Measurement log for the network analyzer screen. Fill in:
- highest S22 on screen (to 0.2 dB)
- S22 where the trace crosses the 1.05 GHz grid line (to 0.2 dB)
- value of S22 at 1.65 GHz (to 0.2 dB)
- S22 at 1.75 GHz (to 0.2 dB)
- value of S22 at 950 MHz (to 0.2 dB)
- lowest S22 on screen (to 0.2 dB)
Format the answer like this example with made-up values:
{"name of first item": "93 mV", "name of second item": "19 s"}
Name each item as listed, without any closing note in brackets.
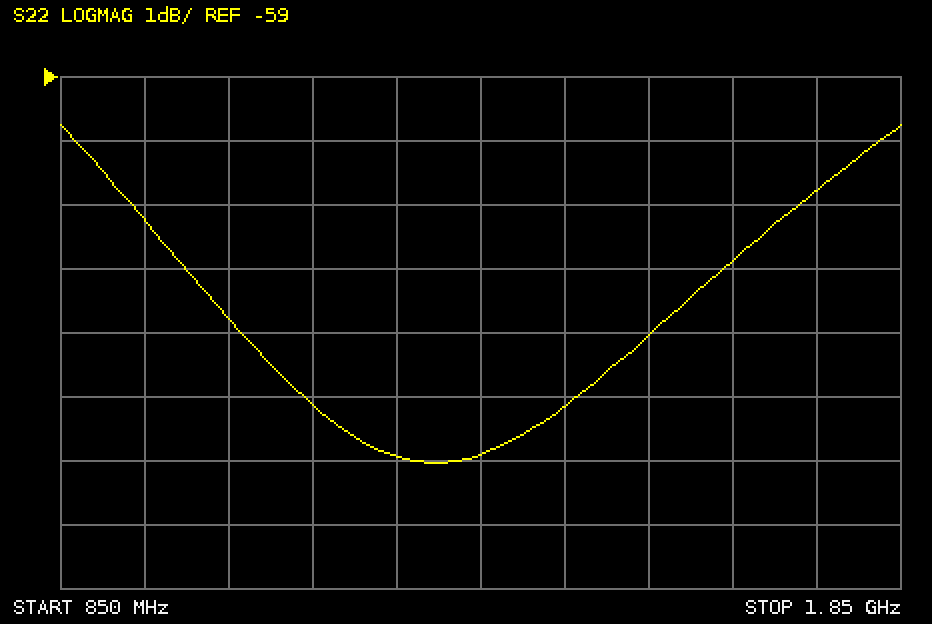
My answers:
{"highest S22 on screen": "-59.8 dB", "S22 where the trace crosses the 1.05 GHz grid line": "-62.8 dB", "value of S22 at 1.65 GHz": "-61.8 dB", "S22 at 1.75 GHz": "-60.8 dB", "value of S22 at 950 MHz": "-61.2 dB", "lowest S22 on screen": "-65.0 dB"}
